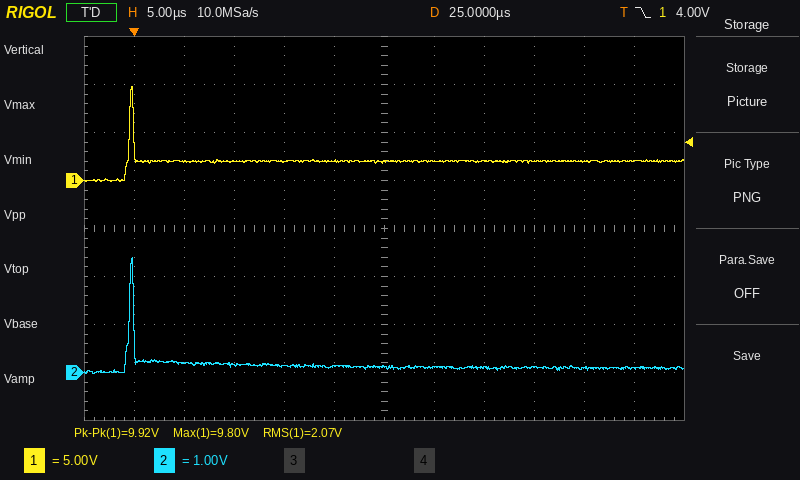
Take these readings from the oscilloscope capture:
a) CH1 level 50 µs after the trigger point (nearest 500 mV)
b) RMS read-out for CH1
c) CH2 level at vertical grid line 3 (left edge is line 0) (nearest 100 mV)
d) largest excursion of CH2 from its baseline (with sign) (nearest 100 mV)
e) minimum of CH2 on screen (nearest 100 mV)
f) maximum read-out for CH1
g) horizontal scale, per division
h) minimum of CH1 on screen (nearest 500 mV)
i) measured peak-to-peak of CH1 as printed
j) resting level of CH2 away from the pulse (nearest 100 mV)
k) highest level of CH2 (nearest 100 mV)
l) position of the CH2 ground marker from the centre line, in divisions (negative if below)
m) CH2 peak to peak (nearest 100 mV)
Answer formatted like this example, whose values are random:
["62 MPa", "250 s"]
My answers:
["2.0 V", "2.07 V", "200 mV", "+2.3 V", "0.0 V", "9.80 V", "5 µs", "0.0 V", "9.92 V", "100 mV", "2.4 V", "-3.0 div", "2.4 V"]
